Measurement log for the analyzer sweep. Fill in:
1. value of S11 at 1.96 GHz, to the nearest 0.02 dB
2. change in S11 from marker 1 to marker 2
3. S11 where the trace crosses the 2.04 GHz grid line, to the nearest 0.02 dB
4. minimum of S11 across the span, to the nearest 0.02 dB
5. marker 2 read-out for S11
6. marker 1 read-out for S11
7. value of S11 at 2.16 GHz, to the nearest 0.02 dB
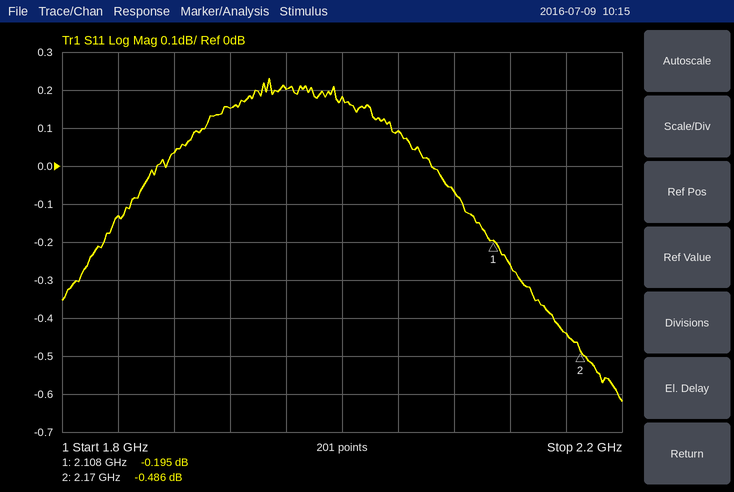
0.20 dB
-0.291 dB
0.10 dB
-0.62 dB
-0.486 dB
-0.195 dB
-0.44 dB
